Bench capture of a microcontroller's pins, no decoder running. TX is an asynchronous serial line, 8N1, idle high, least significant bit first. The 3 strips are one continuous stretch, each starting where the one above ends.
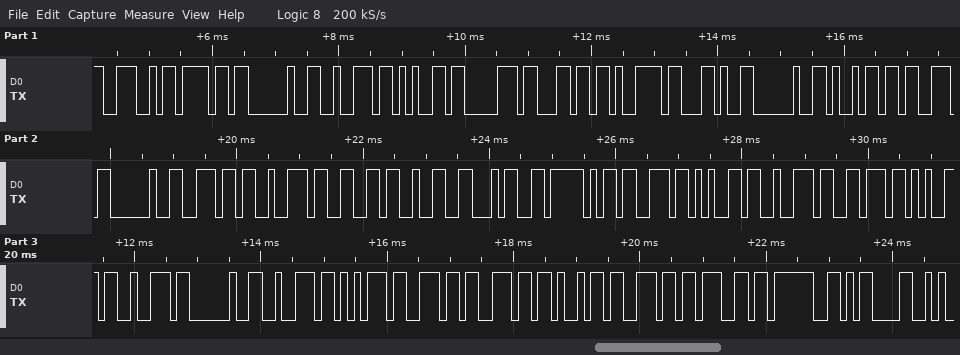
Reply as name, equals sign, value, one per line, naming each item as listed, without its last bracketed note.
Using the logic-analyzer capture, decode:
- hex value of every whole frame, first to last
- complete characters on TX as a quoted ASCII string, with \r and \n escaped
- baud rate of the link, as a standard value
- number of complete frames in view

hex value of every whole frame, first to last = 4E 6F 20 72 65 70 6C 79 2C 20 69 73 20 6E 72 66 32 34 5F 73 65 72 76 65 72 20 72 75 6E 6E 69 6E 67 3F 0D
complete characters on TX as a quoted ASCII string, with \r and \n escaped = "No reply, is nrf24_server running?\r"
baud rate of the link, as a standard value = 9600 baud
number of complete frames in view = 35
